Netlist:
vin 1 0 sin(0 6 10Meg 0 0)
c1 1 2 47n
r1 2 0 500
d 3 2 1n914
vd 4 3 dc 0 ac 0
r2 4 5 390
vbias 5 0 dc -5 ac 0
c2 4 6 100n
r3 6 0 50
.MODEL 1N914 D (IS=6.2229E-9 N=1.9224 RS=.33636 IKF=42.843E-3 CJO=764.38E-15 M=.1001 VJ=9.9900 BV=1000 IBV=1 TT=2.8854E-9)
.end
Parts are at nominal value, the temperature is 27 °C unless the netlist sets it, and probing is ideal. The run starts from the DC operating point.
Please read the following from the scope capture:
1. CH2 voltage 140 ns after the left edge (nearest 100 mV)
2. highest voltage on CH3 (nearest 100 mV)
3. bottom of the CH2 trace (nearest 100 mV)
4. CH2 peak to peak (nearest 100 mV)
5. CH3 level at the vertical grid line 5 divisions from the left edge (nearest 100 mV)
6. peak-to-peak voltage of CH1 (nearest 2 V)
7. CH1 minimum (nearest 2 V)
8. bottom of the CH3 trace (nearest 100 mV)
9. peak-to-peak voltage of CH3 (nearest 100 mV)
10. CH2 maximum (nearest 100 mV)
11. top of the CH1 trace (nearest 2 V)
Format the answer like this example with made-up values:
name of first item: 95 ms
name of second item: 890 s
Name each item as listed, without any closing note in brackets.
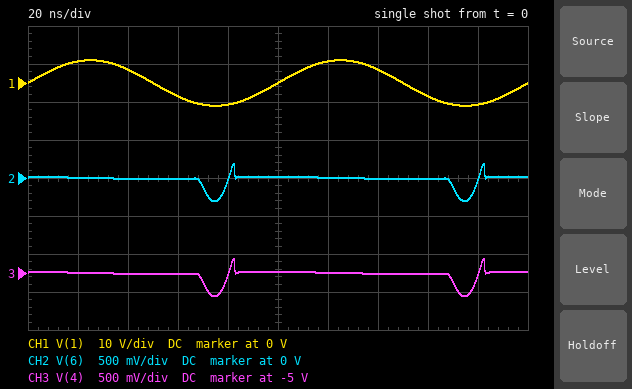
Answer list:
CH2 voltage 140 ns after the left edge: 0 V
highest voltage on CH3: -4.8 V
bottom of the CH2 trace: -300 mV
CH2 peak to peak: 500 mV
CH3 level at the vertical grid line 5 divisions from the left edge: -5.0 V
peak-to-peak voltage of CH1: 12 V
CH1 minimum: -6 V
bottom of the CH3 trace: -5.3 V
peak-to-peak voltage of CH3: 500 mV
CH2 maximum: 200 mV
top of the CH1 trace: 6 V
